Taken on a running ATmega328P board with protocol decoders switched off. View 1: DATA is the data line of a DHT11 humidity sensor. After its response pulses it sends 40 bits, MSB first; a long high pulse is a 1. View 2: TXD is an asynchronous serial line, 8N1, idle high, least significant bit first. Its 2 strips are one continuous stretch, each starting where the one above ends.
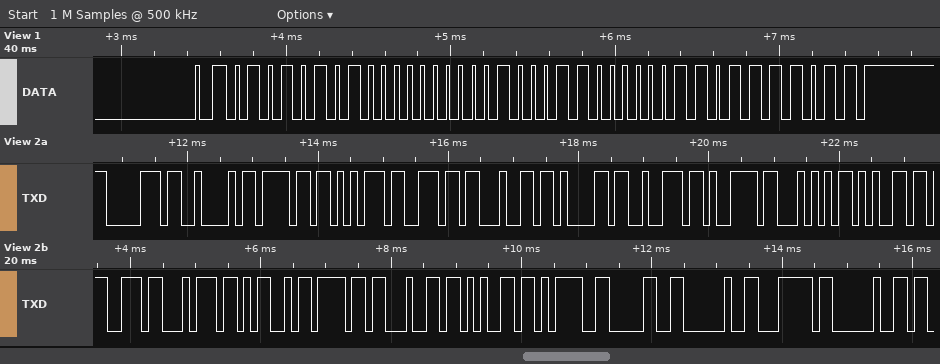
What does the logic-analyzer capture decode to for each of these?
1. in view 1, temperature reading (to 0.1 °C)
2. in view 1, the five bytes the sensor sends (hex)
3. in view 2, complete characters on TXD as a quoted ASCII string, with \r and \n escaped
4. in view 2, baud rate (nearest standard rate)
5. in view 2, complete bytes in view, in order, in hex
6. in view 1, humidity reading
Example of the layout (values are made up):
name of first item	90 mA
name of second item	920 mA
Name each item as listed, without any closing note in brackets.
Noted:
in view 1, temperature reading	35.3 °C
in view 1, the five bytes the sensor sends	55 00 23 03 7B
in view 2, complete characters on TXD as a quoted ASCII string, with \r and \n escaped	"pBoundaryTestMode=0 | "
in view 2, baud rate	9600 baud
in view 2, complete bytes in view, in order, in hex	0x70 0x42 0x6F 0x75 0x6E 0x64 0x61 0x72 0x79 0x54 0x65 0x73 0x74 0x4D 0x6F 0x64 0x65 0x3D 0x30 0x20 0x7C 0x20
in view 1, humidity reading	85 %
